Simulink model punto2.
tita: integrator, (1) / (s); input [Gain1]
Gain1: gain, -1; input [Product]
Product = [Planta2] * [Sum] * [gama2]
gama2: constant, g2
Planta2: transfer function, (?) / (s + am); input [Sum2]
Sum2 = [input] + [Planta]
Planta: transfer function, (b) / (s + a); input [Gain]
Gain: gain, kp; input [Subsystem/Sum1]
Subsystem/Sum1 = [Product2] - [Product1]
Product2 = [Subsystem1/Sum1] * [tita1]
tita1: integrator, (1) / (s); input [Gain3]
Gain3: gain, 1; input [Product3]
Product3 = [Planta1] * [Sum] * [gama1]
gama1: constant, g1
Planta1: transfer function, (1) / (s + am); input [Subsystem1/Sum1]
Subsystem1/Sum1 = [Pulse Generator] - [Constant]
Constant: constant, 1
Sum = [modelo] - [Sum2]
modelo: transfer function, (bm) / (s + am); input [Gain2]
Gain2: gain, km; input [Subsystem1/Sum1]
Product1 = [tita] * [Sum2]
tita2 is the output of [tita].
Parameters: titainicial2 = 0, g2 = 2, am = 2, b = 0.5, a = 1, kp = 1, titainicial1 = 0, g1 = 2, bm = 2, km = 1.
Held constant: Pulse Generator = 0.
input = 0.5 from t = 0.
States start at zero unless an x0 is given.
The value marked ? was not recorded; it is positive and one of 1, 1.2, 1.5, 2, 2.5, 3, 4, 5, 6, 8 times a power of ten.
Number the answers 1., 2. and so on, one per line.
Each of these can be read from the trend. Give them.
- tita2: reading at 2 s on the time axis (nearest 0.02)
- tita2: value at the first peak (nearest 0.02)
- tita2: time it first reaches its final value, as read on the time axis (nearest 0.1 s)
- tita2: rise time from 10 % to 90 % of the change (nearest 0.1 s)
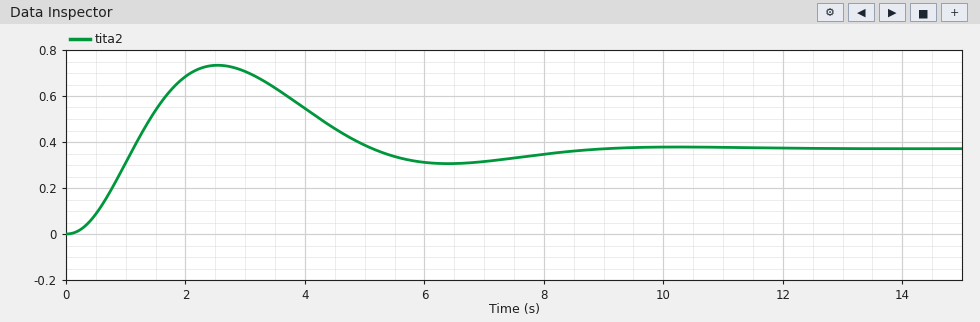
1. 0.68
2. 0.74
3. 1.1 s
4. 0.7 s
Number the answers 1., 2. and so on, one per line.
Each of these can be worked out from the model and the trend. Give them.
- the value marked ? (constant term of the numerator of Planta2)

1. 1
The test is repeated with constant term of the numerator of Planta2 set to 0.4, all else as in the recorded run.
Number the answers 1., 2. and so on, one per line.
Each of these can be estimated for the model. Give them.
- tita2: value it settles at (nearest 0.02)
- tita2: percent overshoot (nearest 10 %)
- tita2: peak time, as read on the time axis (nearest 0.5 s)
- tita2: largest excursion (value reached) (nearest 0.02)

1. 0.20
2. 50 %
3. 2.5 s
4. 0.30
